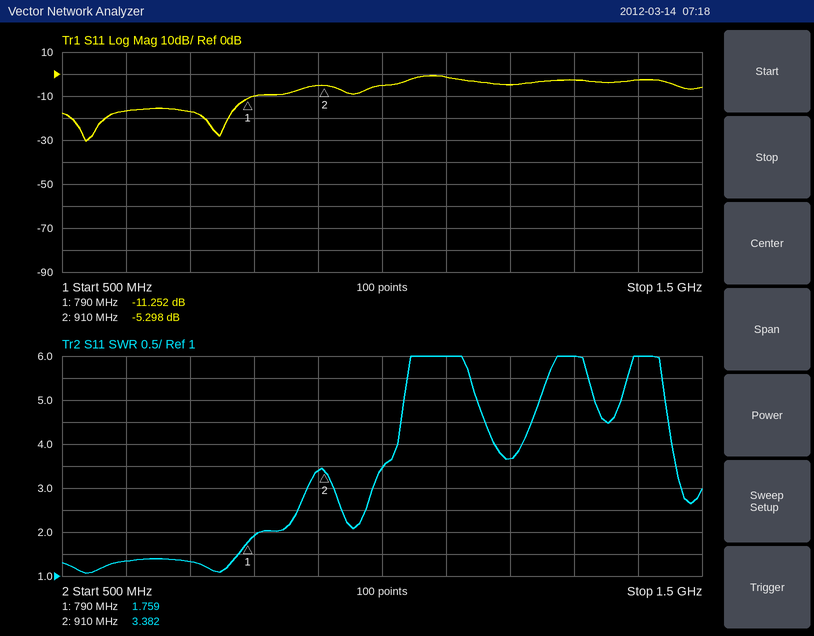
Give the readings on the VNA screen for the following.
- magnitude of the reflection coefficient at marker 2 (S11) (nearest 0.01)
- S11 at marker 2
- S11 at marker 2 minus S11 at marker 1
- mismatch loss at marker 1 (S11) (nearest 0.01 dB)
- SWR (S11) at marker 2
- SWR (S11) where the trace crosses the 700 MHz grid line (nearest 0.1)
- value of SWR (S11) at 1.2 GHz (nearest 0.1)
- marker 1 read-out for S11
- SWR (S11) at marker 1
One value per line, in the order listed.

0.54
-5.298 dB
5.954 dB
0.34 dB
3.382
1.3
3.7
-11.252 dB
1.759
